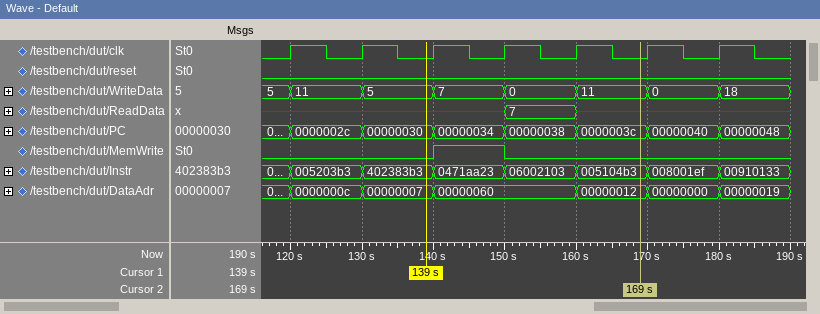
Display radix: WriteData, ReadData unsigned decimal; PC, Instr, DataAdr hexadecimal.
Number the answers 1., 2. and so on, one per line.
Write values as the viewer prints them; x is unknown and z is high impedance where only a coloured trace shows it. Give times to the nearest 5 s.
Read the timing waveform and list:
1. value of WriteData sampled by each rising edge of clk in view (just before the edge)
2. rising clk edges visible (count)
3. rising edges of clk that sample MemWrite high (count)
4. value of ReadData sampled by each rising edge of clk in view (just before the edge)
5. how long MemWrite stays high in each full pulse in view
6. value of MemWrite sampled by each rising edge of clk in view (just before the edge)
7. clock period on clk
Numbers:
1. 5, 11, 5, 7, 0, 11, 0
2. 7
3. 1
4. x, x, x, x, 7, x, x
5. 10 s
6. 0 0 0 1 0 0 0
7. 10 s
